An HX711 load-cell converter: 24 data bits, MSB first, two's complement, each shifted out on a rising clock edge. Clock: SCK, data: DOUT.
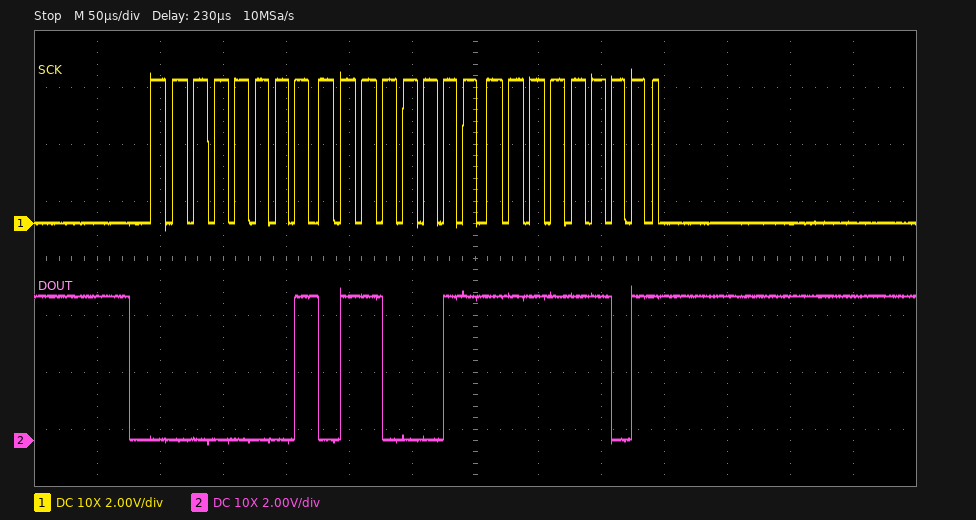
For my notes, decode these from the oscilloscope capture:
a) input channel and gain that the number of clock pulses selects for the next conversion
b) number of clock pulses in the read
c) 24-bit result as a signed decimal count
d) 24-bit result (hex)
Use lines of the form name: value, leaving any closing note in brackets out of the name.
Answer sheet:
input channel and gain that the number of clock pulses selects for the next conversion: channel A, gain 128
number of clock pulses in the read: 25
24-bit result as a signed decimal count: 91133
24-bit result: 0x0163FD
